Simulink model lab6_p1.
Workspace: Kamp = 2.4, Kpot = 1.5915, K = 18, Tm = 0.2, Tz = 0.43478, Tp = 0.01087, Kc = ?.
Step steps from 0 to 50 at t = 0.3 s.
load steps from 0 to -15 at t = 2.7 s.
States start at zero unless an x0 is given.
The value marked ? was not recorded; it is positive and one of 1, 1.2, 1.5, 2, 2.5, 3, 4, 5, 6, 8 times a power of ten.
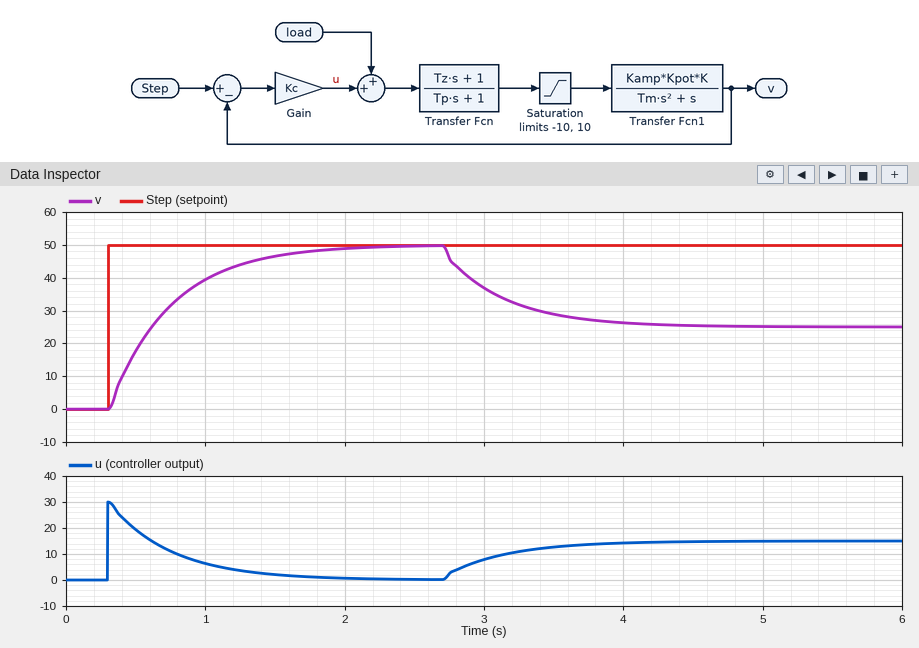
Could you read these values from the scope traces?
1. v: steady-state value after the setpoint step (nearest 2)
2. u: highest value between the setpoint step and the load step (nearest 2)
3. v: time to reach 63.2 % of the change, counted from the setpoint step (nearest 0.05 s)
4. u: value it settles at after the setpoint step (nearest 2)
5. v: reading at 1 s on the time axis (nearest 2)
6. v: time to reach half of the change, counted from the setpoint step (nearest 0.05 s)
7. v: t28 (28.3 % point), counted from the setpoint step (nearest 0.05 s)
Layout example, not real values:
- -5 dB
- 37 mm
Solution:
- 50
- 30
- 0.45 s
- 0
- 40
- 0.30 s
- 0.15 s
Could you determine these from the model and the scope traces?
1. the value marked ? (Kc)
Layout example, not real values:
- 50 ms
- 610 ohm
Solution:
- 0.6
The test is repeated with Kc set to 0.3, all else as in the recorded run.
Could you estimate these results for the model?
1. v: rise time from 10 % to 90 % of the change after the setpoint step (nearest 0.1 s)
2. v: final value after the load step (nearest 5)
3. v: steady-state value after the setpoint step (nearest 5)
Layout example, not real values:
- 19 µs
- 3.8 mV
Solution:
- 1.0 s
- 0
- 50
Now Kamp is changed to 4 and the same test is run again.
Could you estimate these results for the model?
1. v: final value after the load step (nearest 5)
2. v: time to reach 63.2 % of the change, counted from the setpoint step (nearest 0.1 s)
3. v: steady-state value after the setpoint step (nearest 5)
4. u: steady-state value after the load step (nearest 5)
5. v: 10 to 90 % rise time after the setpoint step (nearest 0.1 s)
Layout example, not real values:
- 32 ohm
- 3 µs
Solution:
- 25
- 0.4 s
- 50
- 15
- 1.0 s
